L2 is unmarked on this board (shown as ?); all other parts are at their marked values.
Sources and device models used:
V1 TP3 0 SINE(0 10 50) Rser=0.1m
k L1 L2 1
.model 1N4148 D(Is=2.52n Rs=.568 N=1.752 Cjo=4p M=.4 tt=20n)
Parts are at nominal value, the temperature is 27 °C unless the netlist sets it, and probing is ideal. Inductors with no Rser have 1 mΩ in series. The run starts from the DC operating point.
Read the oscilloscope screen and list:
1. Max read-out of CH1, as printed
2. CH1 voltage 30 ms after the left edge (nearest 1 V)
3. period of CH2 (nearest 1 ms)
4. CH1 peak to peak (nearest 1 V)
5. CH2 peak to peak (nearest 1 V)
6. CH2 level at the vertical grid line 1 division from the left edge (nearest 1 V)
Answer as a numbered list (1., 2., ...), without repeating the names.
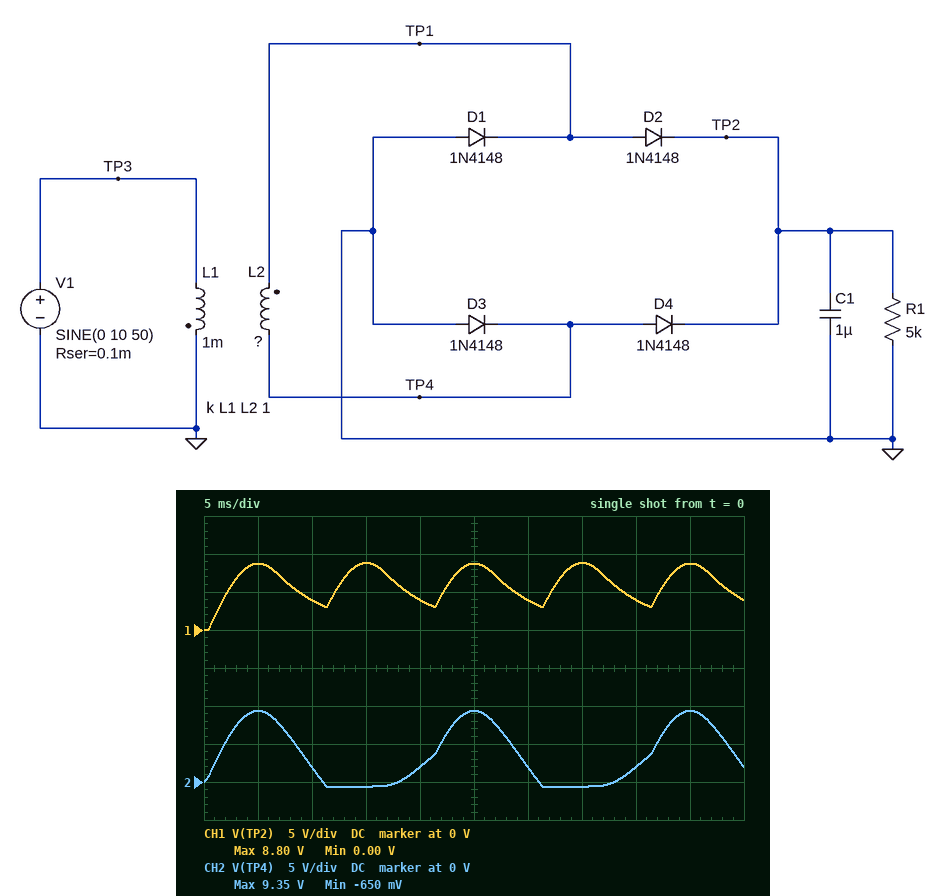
1. 8.80 V
2. 4 V
3. 20 ms
4. 9 V
5. 10 V
6. 9 V
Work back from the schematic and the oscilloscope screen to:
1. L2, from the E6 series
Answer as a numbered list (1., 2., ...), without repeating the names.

1. 1 mH
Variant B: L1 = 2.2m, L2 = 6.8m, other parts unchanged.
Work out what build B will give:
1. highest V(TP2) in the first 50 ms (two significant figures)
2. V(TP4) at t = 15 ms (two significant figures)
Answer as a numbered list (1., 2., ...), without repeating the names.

1. 16 V
2. -640 mV
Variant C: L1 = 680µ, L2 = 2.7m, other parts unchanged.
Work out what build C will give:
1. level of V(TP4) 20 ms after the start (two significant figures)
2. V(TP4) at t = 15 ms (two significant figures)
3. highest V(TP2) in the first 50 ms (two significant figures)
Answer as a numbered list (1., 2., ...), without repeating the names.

1. 4.2 V
2. -650 mV
3. 19 V
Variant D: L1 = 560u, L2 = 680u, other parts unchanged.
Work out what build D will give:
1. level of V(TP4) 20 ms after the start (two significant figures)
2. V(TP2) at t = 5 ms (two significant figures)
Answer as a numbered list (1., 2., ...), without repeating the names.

1. 2.2 V
2. 9.7 V
